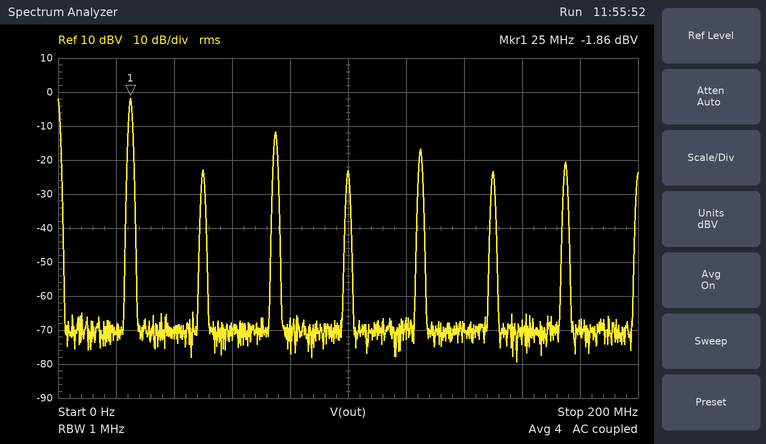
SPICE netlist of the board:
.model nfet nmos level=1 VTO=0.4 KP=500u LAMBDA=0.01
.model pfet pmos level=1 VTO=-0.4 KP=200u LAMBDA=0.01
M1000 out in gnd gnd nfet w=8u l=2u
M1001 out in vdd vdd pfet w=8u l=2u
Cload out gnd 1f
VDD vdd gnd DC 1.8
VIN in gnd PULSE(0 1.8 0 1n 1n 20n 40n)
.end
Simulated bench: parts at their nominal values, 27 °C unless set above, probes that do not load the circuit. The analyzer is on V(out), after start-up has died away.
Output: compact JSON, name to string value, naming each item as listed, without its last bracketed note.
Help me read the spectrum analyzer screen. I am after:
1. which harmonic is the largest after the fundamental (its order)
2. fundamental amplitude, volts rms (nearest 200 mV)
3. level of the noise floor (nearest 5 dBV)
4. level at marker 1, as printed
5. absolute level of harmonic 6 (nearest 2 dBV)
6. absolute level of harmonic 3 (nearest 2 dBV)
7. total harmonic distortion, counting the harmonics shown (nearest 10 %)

{"which harmonic is the largest after the fundamental": "3", "fundamental amplitude, volts rms": "800 mV", "level of the noise floor": "-70 dBV", "level at marker 1, as printed": "-1.86 dBV", "absolute level of harmonic 6": "-24 dBV", "absolute level of harmonic 3": "-12 dBV", "total harmonic distortion, counting the harmonics shown": "40 %"}
